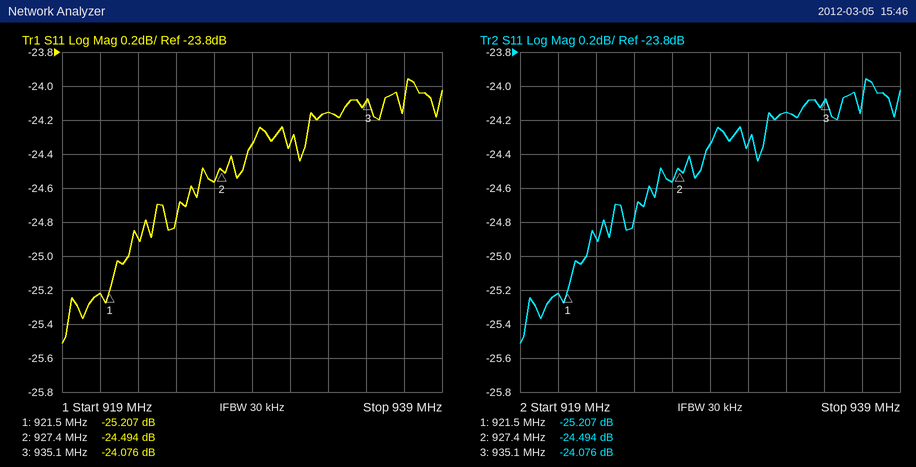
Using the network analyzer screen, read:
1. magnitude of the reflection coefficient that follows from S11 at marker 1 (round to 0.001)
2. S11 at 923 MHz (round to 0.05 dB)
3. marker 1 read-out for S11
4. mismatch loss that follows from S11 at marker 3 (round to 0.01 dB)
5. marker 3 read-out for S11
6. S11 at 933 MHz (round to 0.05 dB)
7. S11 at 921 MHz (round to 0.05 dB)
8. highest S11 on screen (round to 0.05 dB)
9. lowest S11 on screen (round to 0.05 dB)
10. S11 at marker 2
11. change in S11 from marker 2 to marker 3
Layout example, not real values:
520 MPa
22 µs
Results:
0.055
-24.90 dB
-25.207 dB
0.02 dB
-24.076 dB
-24.15 dB
-25.20 dB
-23.95 dB
-25.50 dB
-24.494 dB
0.418 dB
